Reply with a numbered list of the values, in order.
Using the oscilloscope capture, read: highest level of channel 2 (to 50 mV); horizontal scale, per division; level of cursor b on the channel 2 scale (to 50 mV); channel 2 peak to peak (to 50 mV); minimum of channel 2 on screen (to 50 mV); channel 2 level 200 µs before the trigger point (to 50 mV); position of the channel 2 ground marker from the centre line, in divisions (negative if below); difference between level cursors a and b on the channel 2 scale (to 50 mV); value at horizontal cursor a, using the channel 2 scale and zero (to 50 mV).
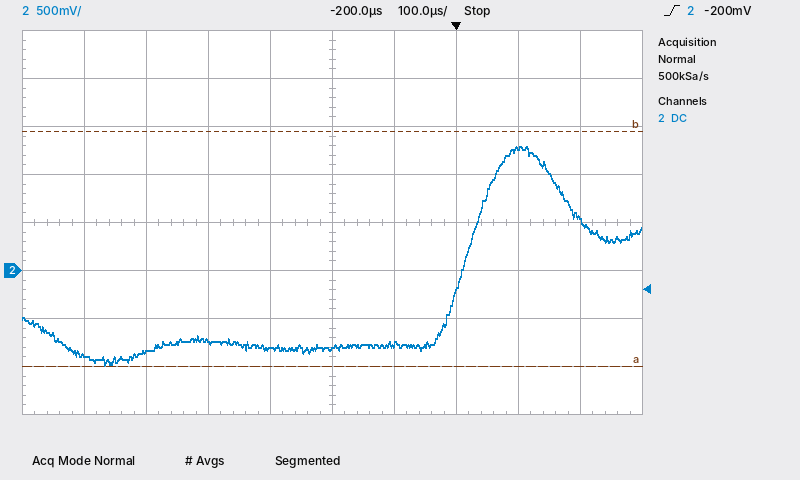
1. 1.30 V
2. 100 µs
3. 1.45 V
4. 2.30 V
5. -1.00 V
6. -800 mV
7. -1.0 div
8. 2.45 V
9. -1.00 V
